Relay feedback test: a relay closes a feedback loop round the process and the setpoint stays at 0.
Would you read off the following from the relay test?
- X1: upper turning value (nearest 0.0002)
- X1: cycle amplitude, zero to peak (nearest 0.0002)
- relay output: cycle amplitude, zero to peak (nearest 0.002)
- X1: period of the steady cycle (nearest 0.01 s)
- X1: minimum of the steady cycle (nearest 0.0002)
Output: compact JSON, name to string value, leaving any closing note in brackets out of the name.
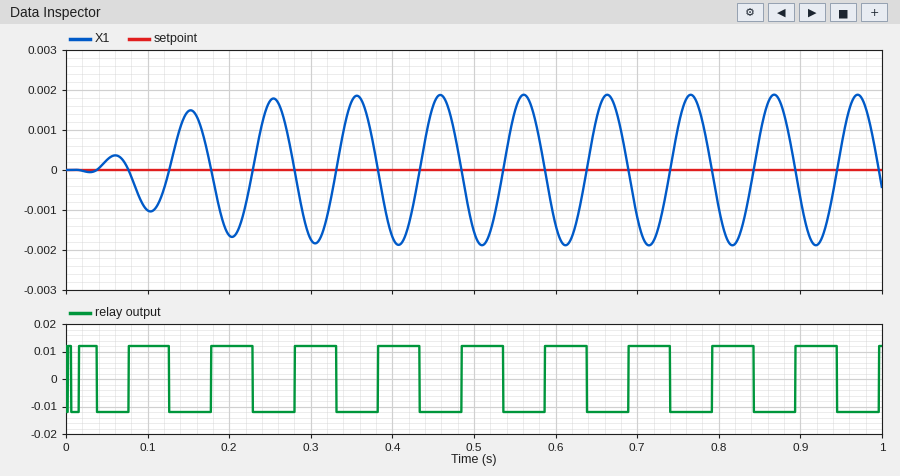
{"X1: upper turning value": "0.0018", "X1: cycle amplitude, zero to peak": "0.0018", "relay output: cycle amplitude, zero to peak": "0.012", "X1: period of the steady cycle": "0.10 s", "X1: minimum of the steady cycle": "-0.0018"}
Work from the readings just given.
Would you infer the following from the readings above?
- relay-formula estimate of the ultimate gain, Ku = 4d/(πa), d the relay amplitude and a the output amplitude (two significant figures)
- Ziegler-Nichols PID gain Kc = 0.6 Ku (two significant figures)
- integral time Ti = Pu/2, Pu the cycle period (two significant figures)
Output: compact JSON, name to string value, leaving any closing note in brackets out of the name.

{"relay-formula estimate of the ultimate gain, Ku = 4d/(πa), d the relay amplitude and a the output amplitude": "8.5", "Ziegler-Nichols PID gain Kc = 0.6 Ku": "5.1", "integral time Ti = Pu/2, Pu the cycle period": "0.050 s"}
